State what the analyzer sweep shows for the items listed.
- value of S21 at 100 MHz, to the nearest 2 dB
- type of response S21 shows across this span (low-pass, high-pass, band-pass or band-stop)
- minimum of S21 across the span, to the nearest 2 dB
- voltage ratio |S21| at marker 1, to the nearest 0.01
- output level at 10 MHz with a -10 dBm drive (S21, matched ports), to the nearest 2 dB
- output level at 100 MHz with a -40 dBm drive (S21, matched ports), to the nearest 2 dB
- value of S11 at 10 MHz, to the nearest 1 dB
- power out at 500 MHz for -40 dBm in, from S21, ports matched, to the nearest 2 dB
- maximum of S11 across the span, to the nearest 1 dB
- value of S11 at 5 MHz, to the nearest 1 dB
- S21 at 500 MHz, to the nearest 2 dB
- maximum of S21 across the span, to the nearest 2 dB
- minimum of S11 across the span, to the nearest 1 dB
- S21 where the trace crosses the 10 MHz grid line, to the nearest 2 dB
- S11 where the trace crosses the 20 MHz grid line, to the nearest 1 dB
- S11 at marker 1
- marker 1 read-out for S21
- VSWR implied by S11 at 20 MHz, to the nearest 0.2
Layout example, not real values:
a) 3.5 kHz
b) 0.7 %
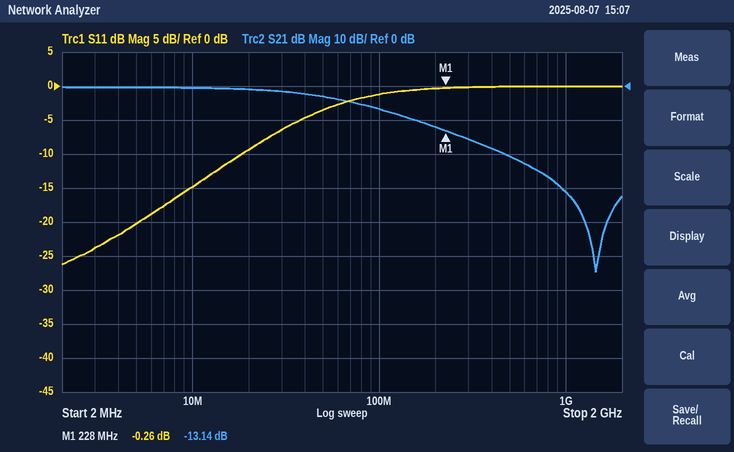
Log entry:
a) -6 dB
b) low-pass
c) -54 dB
d) 0.22
e) -10 dBm
f) -46 dBm
g) -15 dB
h) -60 dBm
i) 0 dB
j) -20 dB
k) -20 dB
l) 0 dB
m) -26 dB
n) 0 dB
o) -9 dB
p) -0.26 dB
q) -13.14 dB
r) 2.0
